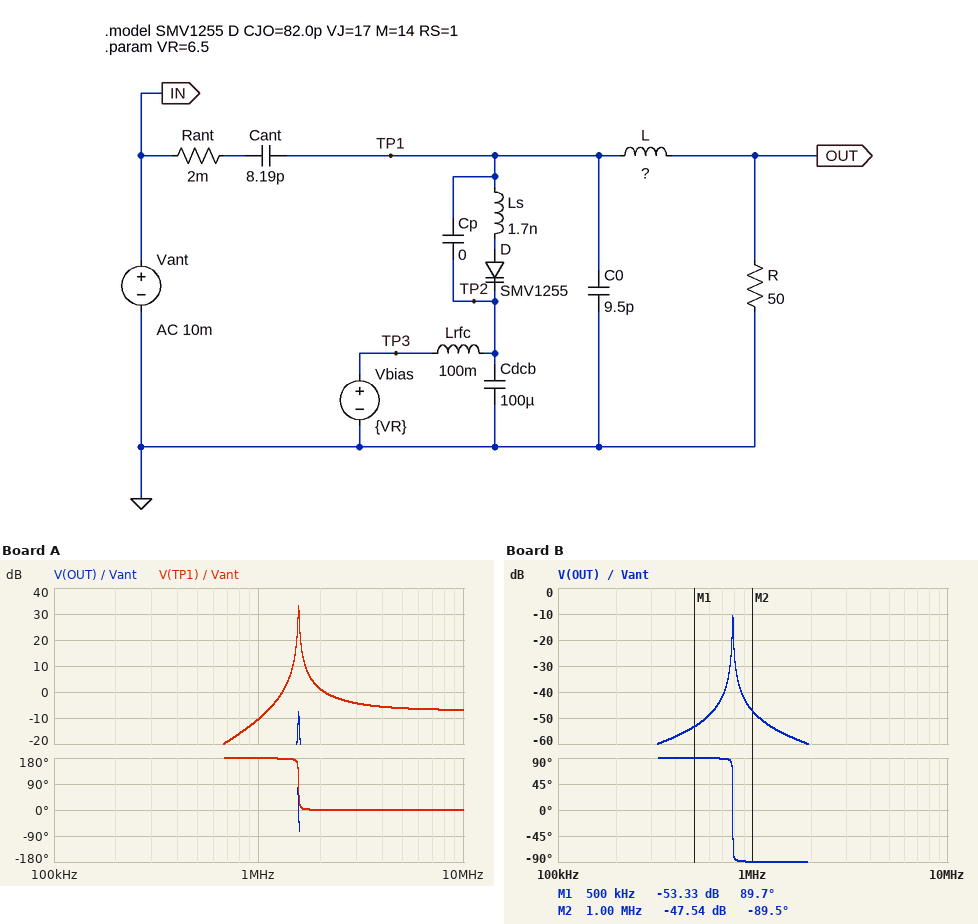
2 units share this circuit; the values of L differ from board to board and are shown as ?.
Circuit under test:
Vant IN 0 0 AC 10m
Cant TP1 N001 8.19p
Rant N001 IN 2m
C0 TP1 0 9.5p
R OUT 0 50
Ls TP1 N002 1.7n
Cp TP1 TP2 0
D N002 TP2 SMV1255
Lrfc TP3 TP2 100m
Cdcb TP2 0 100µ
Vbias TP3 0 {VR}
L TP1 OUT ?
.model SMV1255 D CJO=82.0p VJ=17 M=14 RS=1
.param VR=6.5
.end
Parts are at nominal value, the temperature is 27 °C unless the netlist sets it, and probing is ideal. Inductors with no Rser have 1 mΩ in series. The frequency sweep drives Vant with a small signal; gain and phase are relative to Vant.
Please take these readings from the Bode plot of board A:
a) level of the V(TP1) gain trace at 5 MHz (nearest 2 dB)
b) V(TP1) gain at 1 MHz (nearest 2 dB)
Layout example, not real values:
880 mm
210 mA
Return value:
-6 dB
-10 dB
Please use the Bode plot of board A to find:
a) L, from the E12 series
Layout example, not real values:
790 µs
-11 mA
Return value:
560 µH
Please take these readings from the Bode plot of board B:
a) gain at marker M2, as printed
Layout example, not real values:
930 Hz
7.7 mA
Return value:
-47.54 dB
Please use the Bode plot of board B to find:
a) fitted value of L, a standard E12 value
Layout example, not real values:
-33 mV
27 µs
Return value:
2.2 mH
